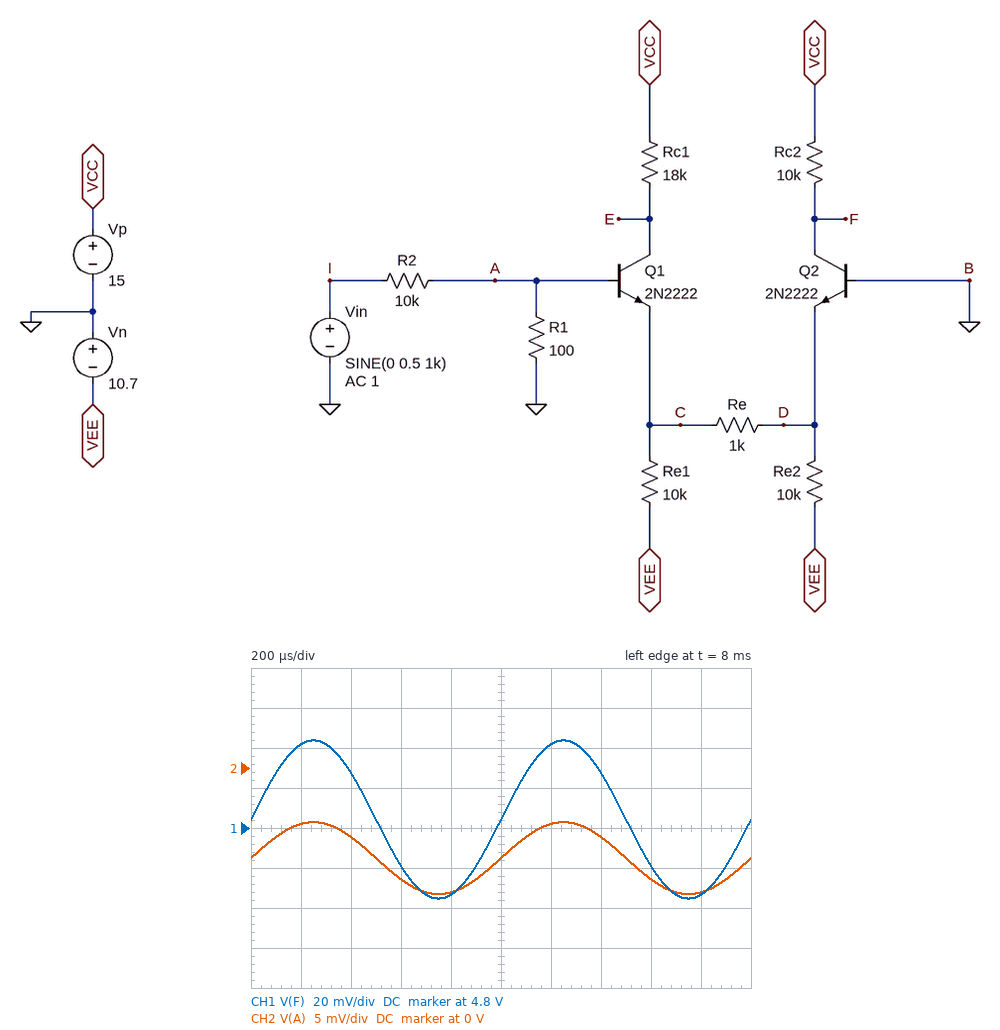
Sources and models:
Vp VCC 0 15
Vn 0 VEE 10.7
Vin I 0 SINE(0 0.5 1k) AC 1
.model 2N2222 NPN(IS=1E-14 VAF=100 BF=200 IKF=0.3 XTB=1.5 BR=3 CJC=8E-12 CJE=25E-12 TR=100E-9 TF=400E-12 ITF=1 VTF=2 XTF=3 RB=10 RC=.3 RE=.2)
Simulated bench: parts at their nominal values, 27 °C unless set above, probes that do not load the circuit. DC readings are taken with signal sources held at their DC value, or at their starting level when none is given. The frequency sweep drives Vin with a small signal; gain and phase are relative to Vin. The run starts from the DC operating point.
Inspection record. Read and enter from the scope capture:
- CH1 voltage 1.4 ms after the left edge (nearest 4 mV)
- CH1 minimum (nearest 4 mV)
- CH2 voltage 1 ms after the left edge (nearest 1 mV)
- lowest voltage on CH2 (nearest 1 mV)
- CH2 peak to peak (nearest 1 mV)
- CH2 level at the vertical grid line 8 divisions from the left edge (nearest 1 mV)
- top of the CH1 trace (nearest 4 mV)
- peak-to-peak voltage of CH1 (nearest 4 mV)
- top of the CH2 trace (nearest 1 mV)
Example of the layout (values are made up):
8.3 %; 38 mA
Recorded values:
4.828 V; 4.764 V; -11 mV; -16 mV; 9 mV; -14 mV; 4.844 V; 80 mV; -7 mV
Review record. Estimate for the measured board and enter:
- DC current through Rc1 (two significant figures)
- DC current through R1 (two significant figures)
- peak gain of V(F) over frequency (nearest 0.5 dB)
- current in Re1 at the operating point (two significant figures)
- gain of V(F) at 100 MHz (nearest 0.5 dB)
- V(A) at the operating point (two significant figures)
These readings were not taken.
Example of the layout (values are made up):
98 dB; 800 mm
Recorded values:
870 µA; 110 µA; -22.0 dB; 1.0 mA; -52.5 dB; -11 mV
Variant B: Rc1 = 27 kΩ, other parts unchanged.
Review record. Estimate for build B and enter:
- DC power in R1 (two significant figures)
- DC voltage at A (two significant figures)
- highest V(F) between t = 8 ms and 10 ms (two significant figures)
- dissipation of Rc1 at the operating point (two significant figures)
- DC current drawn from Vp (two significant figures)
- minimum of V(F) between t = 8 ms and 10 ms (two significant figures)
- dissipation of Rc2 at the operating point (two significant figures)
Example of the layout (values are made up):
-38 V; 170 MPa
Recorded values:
13 µW; -36 mV; 4.5 V; 9.1 mW; 1.6 mA; 4.4 V; 11 mW
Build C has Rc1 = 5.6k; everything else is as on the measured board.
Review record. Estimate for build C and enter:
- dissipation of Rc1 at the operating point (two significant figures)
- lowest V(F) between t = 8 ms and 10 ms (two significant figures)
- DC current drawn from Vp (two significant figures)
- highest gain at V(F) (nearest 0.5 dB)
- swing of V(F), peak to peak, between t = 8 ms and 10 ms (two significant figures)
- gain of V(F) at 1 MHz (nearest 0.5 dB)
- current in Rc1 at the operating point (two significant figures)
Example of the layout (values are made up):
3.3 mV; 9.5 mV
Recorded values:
5.6 mW; 5.0 V; 2.0 mA; -20.5 dB; 93 mV; -21.0 dB; 1.0 mA
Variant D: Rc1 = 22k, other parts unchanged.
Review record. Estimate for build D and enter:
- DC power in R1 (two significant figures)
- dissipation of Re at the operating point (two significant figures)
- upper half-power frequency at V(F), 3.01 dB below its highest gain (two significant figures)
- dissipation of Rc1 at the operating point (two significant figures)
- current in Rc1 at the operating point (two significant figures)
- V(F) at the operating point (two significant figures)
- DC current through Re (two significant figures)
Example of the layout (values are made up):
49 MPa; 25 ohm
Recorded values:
6.0 µW; 1.6 µW; 4.0 MHz; 11 mW; 710 µA; 4.6 V; 40 µA
